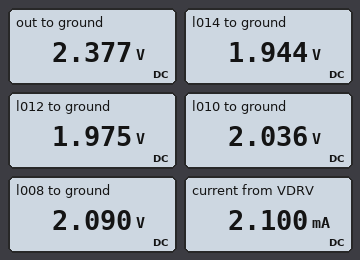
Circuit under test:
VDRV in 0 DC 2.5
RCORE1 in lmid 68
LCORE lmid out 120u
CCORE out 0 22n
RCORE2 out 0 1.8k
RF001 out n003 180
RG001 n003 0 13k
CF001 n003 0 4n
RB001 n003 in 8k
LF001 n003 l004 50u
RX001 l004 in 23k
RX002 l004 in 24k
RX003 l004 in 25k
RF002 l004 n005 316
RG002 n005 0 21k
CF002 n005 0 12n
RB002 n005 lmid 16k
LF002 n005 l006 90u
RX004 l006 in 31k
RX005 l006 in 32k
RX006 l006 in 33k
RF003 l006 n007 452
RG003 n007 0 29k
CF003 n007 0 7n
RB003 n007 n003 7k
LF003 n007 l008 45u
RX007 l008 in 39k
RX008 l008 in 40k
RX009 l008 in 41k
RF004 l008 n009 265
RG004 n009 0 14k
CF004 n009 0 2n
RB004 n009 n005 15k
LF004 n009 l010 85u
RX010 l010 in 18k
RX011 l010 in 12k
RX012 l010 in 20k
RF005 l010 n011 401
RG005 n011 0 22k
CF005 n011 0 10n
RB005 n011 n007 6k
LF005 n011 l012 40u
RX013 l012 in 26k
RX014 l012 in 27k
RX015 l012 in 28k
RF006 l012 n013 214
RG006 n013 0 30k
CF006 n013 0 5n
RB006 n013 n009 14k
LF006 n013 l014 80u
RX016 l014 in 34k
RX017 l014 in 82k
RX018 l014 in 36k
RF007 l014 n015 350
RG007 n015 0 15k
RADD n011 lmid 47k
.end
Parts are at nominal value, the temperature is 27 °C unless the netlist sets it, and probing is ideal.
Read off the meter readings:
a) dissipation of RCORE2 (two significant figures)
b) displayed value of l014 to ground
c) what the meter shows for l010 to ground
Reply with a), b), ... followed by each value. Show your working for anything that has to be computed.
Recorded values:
a) (2.377 V)^2 / 1.8 kΩ = 3.1 mW
b) 1.944 V
c) 2.036 V
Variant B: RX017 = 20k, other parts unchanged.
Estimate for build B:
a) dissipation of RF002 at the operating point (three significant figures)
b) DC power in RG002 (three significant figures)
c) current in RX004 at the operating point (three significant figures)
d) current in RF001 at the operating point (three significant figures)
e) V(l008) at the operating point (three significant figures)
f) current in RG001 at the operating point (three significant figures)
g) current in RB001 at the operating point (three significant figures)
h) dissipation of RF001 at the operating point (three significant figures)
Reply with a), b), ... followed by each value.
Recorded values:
a) 28.8 µW
b) 231 µW
c) 9.66 µA
d) 456 µA
e) 2.10 V
f) 177 µA
g) 25.5 µA
h) 37.4 µW
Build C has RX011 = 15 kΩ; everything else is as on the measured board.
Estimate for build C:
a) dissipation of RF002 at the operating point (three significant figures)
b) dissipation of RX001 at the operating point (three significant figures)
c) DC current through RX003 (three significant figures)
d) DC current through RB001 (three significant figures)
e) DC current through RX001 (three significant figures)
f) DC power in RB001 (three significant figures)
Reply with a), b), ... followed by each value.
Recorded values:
a) 31.1 µW
b) 1.87 µW
c) 8.29 µA
d) 25.9 µA
e) 9.01 µA
f) 5.37 µW
